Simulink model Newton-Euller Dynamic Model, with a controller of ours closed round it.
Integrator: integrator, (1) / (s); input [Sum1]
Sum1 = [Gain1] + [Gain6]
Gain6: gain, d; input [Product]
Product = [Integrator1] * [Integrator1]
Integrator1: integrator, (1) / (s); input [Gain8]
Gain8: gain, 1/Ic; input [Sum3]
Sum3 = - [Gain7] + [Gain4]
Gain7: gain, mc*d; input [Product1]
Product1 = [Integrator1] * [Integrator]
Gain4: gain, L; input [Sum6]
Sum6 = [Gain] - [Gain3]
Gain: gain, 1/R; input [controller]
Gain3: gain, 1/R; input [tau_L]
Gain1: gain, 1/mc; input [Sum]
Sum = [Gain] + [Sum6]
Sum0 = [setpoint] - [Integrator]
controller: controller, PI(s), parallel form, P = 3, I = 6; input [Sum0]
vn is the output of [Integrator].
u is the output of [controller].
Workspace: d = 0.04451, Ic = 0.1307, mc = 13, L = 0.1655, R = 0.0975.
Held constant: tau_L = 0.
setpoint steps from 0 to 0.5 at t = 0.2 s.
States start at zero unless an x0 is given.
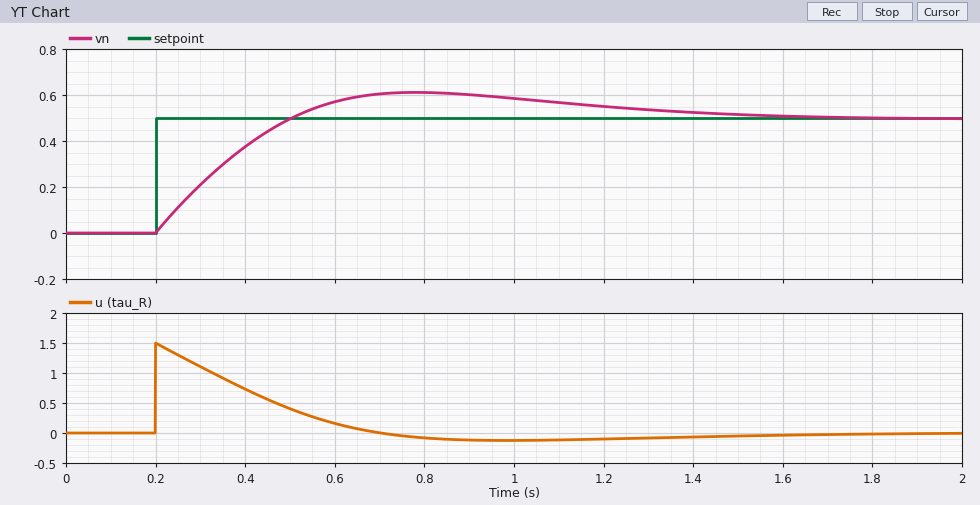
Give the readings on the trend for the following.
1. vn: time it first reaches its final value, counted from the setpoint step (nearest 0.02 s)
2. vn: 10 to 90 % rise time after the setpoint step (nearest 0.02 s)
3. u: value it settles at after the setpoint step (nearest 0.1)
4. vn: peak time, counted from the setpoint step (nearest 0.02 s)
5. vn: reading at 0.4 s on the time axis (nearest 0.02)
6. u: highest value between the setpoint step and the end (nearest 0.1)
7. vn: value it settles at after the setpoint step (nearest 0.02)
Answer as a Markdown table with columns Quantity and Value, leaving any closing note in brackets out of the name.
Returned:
| Quantity | Value |
|---|---|
| vn: time it first reaches its final value, counted from the setpoint step | 0.30 s |
| vn: 10 to 90 % rise time after the setpoint step | 0.24 s |
| u: value it settles at after the setpoint step | 0.0 |
| vn: peak time, counted from the setpoint step | 0.58 s |
| vn: reading at 0.4 s on the time axis | 0.38 |
| u: highest value between the setpoint step and the end | 1.5 |
| vn: value it settles at after the setpoint step | 0.50 |
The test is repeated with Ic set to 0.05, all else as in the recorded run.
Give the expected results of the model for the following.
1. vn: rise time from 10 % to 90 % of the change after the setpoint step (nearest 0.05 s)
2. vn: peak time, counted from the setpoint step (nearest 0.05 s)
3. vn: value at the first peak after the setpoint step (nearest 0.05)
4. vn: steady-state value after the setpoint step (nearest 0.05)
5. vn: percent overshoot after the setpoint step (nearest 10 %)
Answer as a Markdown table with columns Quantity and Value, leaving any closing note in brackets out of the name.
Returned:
| Quantity | Value |
|---|---|
| vn: rise time from 10 % to 90 % of the change after the setpoint step | 0.20 s |
| vn: peak time, counted from the setpoint step | 0.45 s |
| vn: value at the first peak after the setpoint step | 0.60 |
| vn: steady-state value after the setpoint step | 0.50 |
| vn: percent overshoot after the setpoint step | 20 % |
